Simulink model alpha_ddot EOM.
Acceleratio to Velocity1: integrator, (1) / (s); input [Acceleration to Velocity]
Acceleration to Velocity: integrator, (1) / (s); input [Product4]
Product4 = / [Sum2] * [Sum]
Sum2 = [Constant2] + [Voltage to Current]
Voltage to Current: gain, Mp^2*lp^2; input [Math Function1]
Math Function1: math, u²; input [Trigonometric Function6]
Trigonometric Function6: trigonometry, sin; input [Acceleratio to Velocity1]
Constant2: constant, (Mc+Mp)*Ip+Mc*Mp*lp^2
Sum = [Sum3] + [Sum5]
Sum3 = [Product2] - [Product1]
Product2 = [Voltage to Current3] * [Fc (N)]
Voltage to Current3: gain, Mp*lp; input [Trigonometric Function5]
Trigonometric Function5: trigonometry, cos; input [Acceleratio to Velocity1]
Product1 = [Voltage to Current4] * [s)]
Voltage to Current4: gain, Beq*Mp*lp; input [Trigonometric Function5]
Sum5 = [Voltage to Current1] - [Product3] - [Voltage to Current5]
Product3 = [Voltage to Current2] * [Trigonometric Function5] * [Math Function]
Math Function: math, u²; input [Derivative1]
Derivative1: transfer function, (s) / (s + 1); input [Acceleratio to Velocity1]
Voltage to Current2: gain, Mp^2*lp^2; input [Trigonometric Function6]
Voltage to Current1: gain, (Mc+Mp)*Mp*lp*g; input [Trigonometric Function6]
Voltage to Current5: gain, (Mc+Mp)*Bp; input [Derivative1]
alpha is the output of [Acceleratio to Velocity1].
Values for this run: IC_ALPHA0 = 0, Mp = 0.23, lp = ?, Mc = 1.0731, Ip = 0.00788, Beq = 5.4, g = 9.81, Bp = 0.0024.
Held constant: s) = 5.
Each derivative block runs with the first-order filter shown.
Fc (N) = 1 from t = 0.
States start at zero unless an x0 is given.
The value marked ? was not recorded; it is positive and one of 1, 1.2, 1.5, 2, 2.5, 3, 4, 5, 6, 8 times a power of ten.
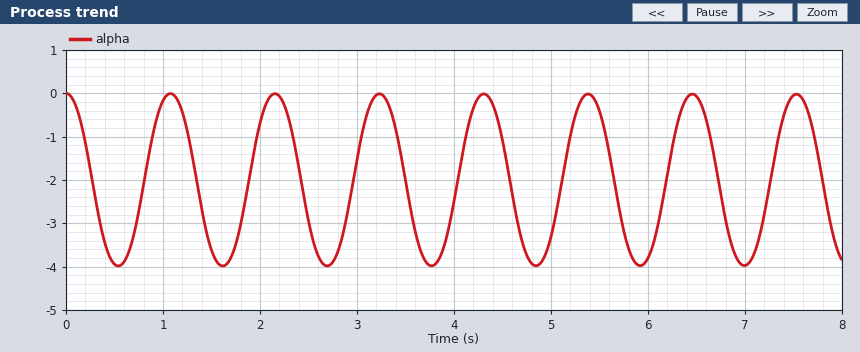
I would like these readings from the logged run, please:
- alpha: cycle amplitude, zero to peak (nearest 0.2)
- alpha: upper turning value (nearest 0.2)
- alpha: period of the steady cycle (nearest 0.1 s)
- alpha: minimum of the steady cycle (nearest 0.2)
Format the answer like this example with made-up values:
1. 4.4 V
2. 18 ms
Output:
1. 2.0
2. 0.0
3. 1.1 s
4. -4.0
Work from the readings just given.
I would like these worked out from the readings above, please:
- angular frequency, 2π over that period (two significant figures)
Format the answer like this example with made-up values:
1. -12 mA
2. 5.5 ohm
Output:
1. 5.7 rad/s
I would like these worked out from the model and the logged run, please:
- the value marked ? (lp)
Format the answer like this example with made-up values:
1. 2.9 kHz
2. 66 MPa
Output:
1. 0.3
